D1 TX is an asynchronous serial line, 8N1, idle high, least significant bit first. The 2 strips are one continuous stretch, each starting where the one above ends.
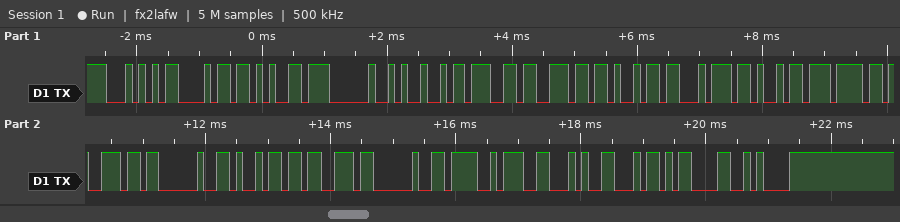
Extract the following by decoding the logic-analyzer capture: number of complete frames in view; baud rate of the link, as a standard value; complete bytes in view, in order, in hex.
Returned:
21
9600 baud
54 68 65 20 49 67 6E 69 74 69 6F 6E 20 69 73 20 4F 46 46 0D 0A
